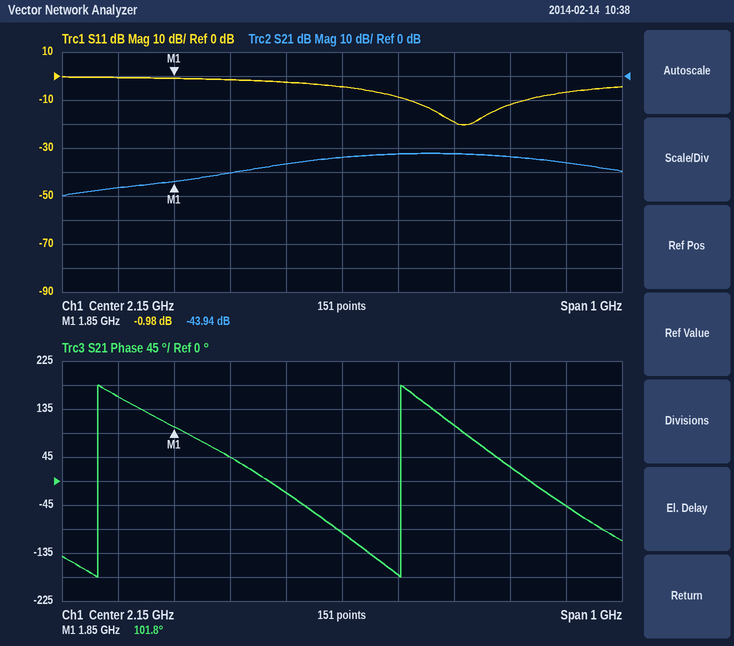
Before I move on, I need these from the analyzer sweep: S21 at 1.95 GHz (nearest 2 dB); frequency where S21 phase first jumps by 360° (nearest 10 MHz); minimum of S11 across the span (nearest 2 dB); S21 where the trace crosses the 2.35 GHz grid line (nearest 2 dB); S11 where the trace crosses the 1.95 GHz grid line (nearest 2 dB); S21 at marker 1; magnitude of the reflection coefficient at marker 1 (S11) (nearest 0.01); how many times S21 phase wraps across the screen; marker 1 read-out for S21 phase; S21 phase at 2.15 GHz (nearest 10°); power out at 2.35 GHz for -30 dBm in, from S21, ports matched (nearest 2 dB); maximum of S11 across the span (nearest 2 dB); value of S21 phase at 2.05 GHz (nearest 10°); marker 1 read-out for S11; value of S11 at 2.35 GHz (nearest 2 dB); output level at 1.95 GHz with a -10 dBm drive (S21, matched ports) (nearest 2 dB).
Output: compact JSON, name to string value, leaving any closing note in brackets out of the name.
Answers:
{"S21 at 1.95 GHz": "-40 dB", "frequency where S21 phase first jumps by 360°": "1.71 GHz", "minimum of S11 across the span": "-20 dB", "S21 where the trace crosses the 2.35 GHz grid line": "-32 dB", "S11 where the trace crosses the 1.95 GHz grid line": "-2 dB", "S21 at marker 1": "-43.94 dB", "magnitude of the reflection coefficient at marker 1 (S11)": "0.89", "how many times S21 phase wraps across the screen": "2", "marker 1 read-out for S21 phase": "101.8°", "S21 phase at 2.15 GHz": "-100°", "power out at 2.35 GHz for -30 dBm in, from S21, ports matched": "-62 dBm", "maximum of S11 across the span": "0 dB", "value of S21 phase at 2.05 GHz": "-20°", "marker 1 read-out for S11": "-0.98 dB", "value of S11 at 2.35 GHz": "-20 dB", "output level at 1.95 GHz with a -10 dBm drive (S21, matched ports)": "-50 dBm"}
